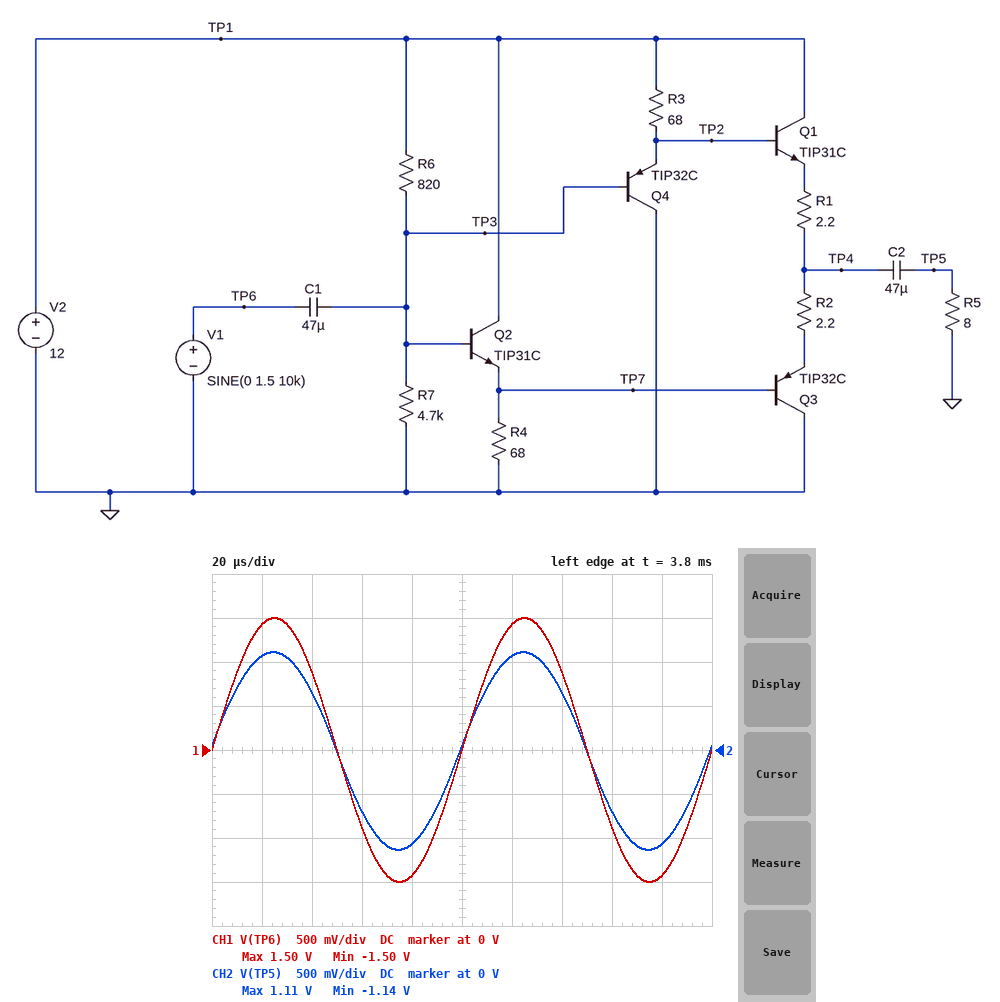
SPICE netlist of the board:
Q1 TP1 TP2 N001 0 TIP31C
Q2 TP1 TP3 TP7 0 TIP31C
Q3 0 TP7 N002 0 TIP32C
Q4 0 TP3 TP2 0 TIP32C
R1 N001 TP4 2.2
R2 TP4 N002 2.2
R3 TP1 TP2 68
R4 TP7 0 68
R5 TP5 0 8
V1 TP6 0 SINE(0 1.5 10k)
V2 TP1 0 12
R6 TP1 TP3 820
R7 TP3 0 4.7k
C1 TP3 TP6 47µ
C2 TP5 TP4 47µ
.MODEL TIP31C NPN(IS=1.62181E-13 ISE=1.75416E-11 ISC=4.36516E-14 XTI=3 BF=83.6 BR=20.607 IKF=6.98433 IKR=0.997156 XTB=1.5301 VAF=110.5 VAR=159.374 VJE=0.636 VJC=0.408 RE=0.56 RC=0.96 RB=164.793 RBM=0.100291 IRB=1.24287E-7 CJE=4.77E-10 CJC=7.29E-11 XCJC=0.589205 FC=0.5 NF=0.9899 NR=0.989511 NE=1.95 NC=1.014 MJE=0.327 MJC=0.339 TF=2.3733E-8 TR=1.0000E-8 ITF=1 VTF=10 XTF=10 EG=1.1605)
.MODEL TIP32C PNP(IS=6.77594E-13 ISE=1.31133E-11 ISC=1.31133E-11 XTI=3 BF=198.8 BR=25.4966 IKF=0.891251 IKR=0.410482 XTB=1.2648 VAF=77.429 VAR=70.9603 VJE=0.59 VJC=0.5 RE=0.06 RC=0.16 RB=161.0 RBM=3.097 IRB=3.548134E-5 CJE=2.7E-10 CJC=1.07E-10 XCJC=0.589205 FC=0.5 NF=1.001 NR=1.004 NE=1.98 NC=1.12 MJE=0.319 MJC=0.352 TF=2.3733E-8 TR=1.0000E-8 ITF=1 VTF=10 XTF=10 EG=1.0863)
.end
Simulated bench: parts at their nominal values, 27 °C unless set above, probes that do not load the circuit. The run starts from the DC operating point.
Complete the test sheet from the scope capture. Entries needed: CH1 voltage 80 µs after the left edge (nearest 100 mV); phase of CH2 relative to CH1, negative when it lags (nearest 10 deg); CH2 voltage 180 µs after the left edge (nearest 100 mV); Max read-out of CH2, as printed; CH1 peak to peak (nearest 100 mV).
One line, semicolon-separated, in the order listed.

-1.4 V; 0 deg; -1.1 V; 1.11 V; 3.0 V
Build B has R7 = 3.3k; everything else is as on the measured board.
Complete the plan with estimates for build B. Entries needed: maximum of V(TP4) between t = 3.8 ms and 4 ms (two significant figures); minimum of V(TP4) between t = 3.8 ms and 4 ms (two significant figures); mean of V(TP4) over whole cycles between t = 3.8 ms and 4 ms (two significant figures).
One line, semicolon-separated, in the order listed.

9.8 V; 7.6 V; 8.7 V
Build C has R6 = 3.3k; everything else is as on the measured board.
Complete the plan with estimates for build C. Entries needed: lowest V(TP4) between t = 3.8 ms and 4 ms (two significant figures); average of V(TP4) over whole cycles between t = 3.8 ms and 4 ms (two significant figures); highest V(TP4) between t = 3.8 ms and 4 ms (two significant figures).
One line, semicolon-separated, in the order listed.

4.9 V; 6.0 V; 7.1 V
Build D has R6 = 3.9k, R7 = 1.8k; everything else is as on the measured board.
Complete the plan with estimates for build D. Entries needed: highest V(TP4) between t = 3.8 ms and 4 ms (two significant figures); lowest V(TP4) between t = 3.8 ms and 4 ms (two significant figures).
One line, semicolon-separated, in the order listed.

5.0 V; 2.7 V
